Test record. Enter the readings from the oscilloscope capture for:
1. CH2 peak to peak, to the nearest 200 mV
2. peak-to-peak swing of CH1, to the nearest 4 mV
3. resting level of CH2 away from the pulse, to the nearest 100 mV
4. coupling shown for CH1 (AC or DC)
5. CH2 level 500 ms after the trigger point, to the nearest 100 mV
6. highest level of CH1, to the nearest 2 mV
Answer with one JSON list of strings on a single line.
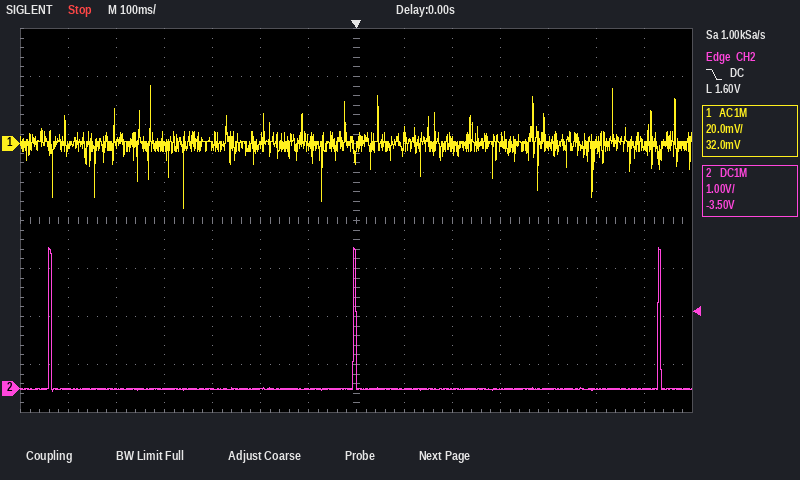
["3.0 V", "52 mV", "0.0 V", "AC", "0.0 V", "24 mV"]
